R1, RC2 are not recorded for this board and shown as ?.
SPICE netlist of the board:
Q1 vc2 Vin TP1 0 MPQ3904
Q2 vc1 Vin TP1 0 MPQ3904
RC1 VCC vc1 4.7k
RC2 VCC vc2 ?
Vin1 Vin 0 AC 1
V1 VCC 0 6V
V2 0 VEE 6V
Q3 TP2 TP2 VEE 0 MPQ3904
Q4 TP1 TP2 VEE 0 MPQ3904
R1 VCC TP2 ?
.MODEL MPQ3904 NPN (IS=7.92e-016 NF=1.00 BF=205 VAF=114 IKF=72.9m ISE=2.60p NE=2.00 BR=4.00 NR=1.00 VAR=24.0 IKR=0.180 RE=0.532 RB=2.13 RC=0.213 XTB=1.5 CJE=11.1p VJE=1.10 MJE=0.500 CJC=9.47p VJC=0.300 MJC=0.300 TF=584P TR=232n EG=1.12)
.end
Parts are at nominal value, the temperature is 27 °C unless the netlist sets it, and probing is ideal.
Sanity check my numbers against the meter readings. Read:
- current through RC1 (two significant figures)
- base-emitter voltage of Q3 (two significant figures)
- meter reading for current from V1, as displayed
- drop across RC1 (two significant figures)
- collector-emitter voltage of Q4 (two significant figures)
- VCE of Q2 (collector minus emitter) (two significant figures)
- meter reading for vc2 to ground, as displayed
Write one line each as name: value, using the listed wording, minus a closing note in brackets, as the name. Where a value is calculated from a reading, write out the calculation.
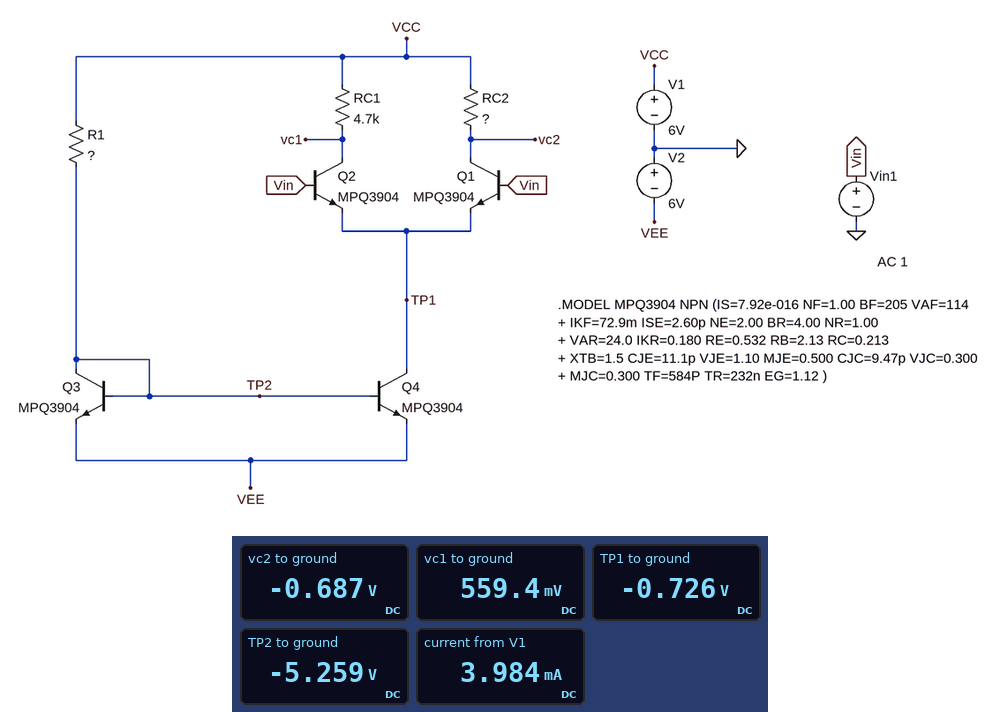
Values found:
current through RC1: (6 V - 559.4 mV) / 4.7 kΩ = 1.2 mA
base-emitter voltage of Q3: -5.259 V - (-6 V) = 740 mV
meter reading for current from V1, as displayed: 3.984 mA
drop across RC1: 6 V - 559.4 mV = 5.4 V
collector-emitter voltage of Q4: -726 mV - (-6 V) = 5.3 V
VCE of Q2 (collector minus emitter): 559.4 mV - (-726 mV) = 1.3 V
meter reading for vc2 to ground, as displayed: -0.687 V
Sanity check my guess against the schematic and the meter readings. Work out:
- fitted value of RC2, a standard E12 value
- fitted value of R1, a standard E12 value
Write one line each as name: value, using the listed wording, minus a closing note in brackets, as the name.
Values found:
fitted value of RC2, a standard E12 value: 8.2 kΩ
fitted value of R1, a standard E12 value: 5.6 kΩ
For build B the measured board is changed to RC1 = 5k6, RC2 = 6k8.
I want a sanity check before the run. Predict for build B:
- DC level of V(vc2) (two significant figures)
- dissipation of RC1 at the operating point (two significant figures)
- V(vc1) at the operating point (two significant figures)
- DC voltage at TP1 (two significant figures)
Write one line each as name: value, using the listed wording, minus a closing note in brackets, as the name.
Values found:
DC level of V(vc2): -650 mV
dissipation of RC1 at the operating point: 6.2 mW
V(vc1) at the operating point: 110 mV
DC voltage at TP1: -720 mV
